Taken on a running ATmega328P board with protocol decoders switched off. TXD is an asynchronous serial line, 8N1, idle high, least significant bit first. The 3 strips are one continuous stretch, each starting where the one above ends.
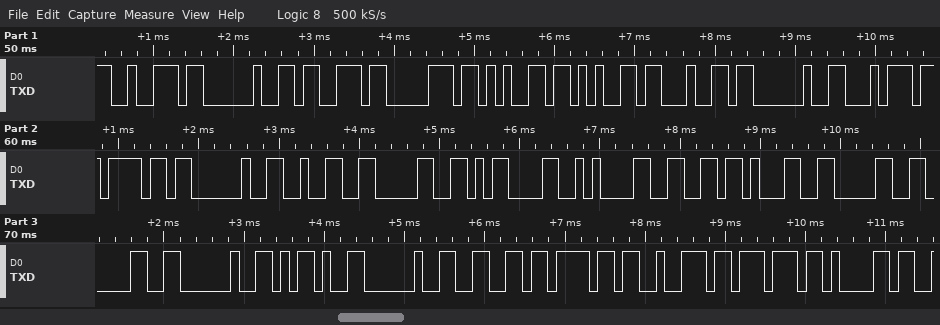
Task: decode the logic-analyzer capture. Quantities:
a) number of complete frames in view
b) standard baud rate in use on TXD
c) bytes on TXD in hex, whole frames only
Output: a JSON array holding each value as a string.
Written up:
["27", "9600 baud", "72 20 73 70 65 65 64 20 74 6F 20 32 30 0D 0A 66 31 30 30 20 2D 20 66 6F 72 77 61"]
